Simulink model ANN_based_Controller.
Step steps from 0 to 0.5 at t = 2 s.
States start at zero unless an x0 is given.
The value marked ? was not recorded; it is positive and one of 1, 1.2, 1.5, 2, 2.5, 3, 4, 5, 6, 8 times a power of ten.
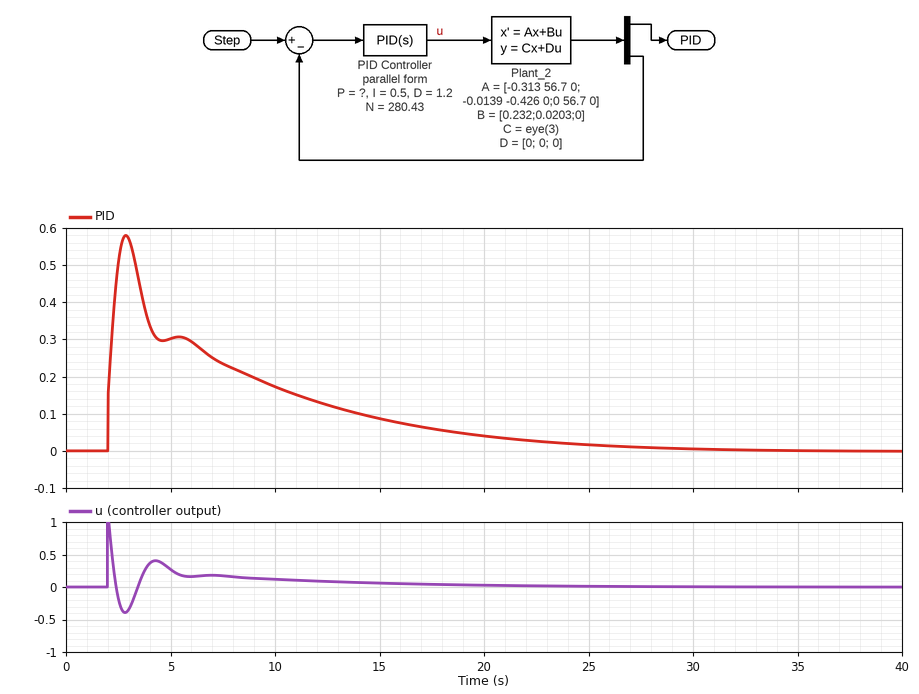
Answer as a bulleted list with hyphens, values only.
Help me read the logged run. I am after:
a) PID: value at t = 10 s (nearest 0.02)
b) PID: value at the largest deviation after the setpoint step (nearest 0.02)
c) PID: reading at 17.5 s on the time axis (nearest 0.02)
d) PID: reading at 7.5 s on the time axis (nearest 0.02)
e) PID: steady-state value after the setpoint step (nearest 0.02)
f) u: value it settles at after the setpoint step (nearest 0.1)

- 0.18
- 0.58
- 0.06
- 0.24
- 0.00
- 0.0
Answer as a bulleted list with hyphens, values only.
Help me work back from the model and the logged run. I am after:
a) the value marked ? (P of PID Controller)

- 4
